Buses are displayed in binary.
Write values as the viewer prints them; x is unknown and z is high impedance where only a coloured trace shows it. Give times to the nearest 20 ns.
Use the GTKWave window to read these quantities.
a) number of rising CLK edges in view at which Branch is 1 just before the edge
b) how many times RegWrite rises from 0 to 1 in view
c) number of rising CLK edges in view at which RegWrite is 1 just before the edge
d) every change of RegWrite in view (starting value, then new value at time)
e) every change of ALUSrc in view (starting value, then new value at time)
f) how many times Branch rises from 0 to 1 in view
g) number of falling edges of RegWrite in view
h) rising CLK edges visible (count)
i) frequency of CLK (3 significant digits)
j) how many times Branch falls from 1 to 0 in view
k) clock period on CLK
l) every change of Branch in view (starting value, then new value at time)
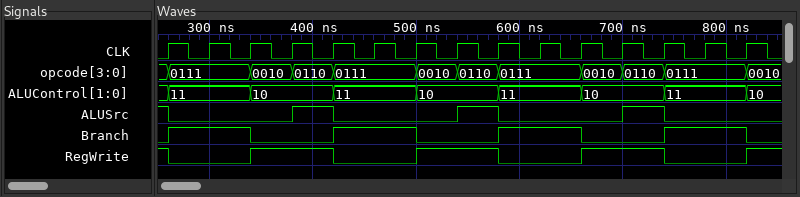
8
4
7
1, 0 at 260 ns, 1 at 340 ns, 0 at 420 ns, 1 at 500 ns, 0 at 580 ns, 1 at 660 ns, 0 at 740 ns, 1 at 820 ns
1, 0 at 260 ns, 1 at 380 ns, 0 at 420 ns, 1 at 540 ns, 0 at 580 ns, 1 at 700 ns, 0 at 740 ns
4
4
15
25.0 MHz
4
40 ns
0, 1 at 260 ns, 0 at 340 ns, 1 at 420 ns, 0 at 500 ns, 1 at 580 ns, 0 at 660 ns, 1 at 740 ns, 0 at 820 ns
